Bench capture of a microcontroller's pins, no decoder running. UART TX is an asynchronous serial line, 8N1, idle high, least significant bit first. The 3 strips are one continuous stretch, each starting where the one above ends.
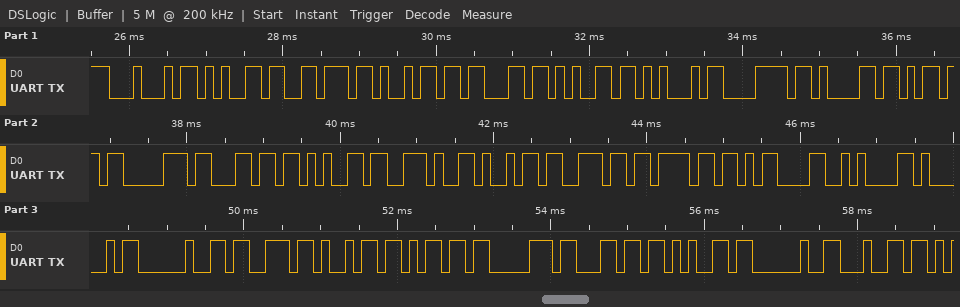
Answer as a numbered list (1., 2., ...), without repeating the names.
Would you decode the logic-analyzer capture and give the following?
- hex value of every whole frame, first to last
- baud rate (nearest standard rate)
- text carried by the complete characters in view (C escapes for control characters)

1. 44 65 76 69 63 65 45 78 61 6D 70 6C 65 2E 69 6E 6F 0D 0A 41 20 73 69 6D 70 6C 65 20 64
2. 9600 baud
3. "DeviceExample.ino\r\nA simple d"
